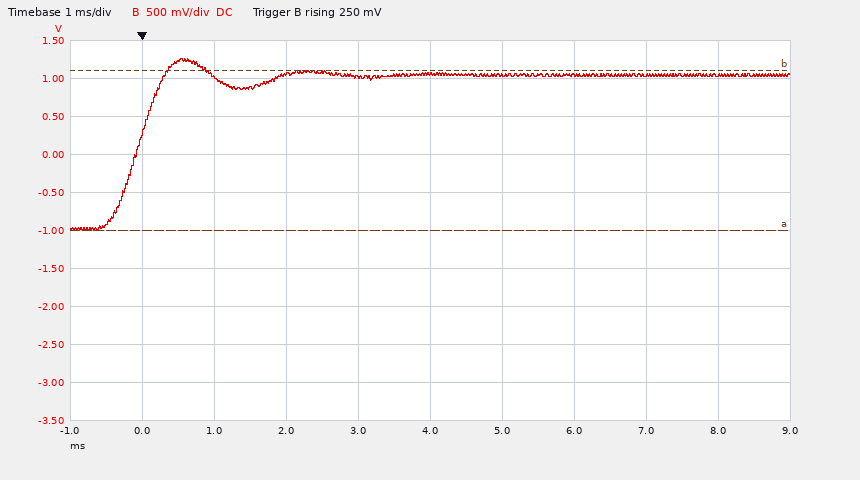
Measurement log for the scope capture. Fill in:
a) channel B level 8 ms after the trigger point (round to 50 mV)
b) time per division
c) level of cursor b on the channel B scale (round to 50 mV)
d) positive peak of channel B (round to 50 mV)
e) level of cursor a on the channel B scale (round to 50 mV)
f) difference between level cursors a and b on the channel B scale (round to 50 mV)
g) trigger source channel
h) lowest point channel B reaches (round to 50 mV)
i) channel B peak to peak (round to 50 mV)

1.05 V
1 ms
1.10 V
1.25 V
-1.00 V
2.10 V
channel B
-1.00 V
2.25 V
